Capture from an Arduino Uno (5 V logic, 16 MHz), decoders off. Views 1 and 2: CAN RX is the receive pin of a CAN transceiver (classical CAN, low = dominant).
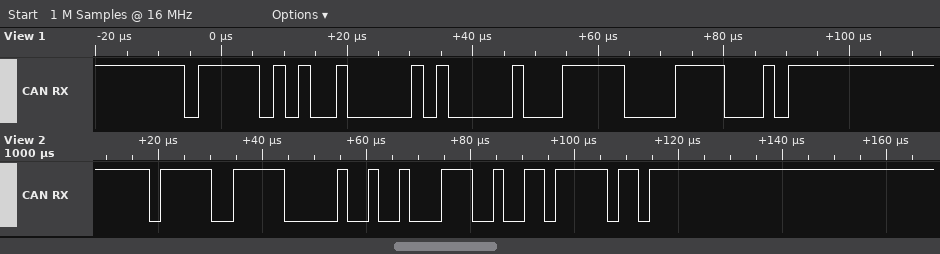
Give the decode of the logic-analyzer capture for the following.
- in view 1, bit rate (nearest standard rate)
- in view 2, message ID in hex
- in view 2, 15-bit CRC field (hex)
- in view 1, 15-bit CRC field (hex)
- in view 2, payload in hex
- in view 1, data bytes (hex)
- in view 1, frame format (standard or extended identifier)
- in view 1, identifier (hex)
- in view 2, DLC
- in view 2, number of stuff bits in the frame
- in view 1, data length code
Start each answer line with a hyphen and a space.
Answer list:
- 500 kbit/s
- 0x7DF
- 0x49BF
- 0x7C78
- 23
- 00
- standard
- 0x7E9
- 1
- 4
- 1
